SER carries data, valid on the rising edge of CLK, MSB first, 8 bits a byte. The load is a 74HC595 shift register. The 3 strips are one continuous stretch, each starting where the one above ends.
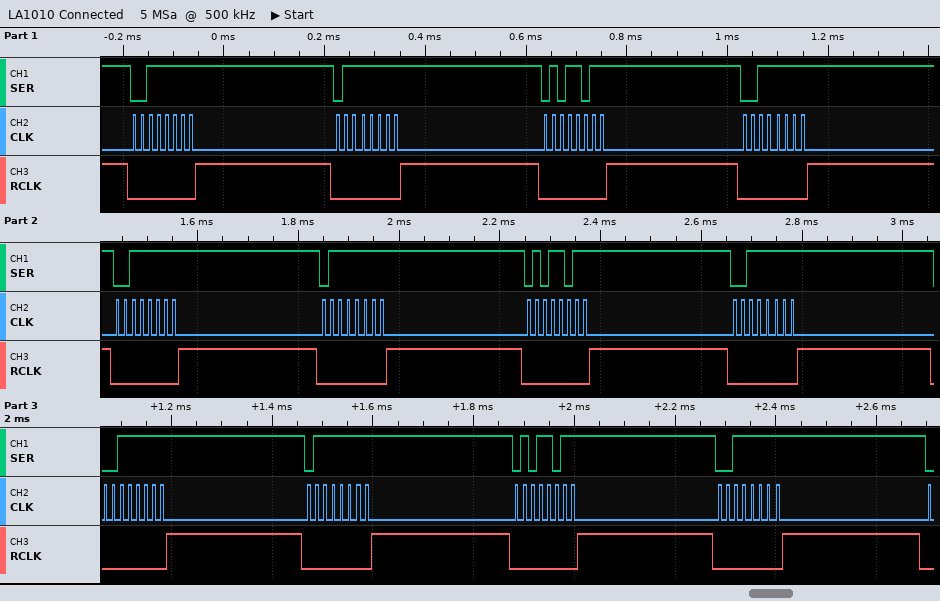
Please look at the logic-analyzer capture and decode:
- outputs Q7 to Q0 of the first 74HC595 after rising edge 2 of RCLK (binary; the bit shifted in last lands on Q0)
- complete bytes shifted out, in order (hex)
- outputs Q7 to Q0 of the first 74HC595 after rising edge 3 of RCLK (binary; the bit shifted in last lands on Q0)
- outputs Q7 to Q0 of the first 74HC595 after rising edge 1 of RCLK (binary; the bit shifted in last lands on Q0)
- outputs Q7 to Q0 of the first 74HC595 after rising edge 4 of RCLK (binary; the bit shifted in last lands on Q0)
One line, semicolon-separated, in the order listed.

01111111; 0x3F 0x7F 0x5B 0x3F 0x3F 0x7F 0x5B 0x3F 0x3F 0x7F 0x5B 0x3F; 01011011; 00111111; 00111111
